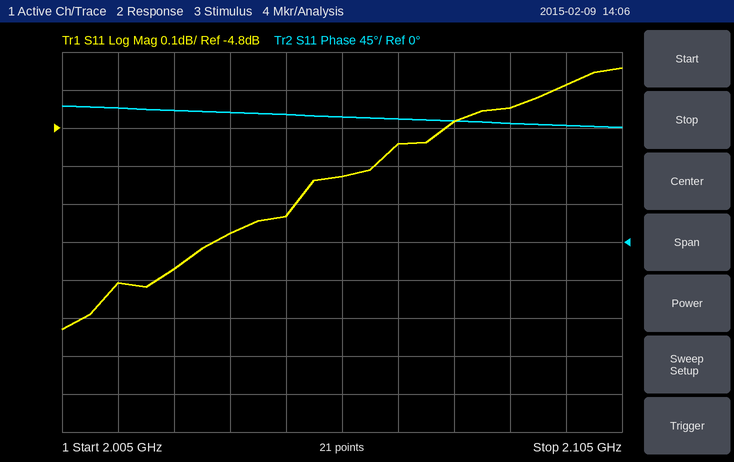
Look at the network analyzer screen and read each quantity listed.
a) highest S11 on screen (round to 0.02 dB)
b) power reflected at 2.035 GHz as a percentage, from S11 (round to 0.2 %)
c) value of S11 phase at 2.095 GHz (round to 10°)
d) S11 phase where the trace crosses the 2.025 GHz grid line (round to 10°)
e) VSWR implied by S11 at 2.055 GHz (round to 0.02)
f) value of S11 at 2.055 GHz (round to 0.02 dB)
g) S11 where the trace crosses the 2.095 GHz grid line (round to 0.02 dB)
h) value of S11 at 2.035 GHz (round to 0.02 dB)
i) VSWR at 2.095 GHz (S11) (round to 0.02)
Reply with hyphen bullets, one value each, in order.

- -4.64 dB
- 31.0 %
- 140°
- 160°
- 3.62
- -4.92 dB
- -4.68 dB
- -5.08 dB
- 3.80
